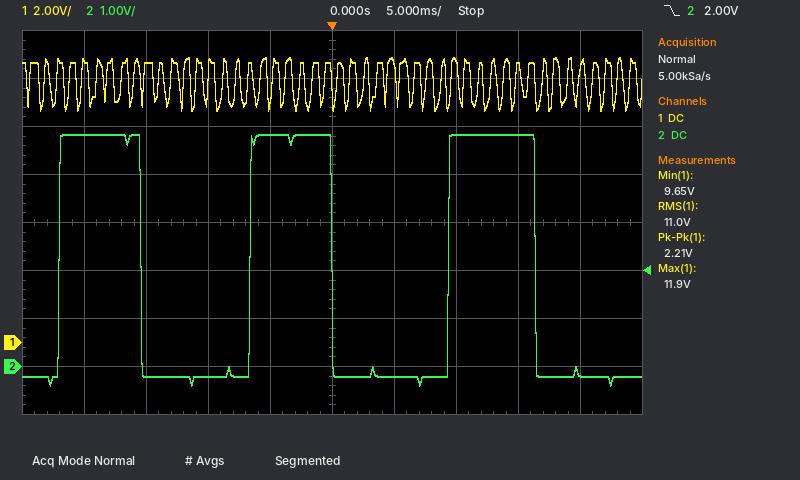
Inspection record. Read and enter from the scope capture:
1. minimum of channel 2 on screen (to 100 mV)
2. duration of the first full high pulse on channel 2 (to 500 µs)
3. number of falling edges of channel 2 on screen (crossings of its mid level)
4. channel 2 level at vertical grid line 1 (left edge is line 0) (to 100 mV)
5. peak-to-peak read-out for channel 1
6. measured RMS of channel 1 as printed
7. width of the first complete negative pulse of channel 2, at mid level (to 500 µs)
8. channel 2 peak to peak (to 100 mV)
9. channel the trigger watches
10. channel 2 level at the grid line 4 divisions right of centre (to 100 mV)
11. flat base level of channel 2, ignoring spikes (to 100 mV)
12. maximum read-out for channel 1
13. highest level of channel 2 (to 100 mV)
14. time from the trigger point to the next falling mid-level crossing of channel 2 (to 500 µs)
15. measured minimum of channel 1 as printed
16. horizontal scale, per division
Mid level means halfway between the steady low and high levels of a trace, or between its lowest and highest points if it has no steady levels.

-400 mV
6.5 ms
3
4.8 V
2.21 V
11.0 V
9.0 ms
5.2 V
channel 2
-100 mV
-200 mV
11.9 V
4.8 V
16.5 ms
9.65 V
5 ms
